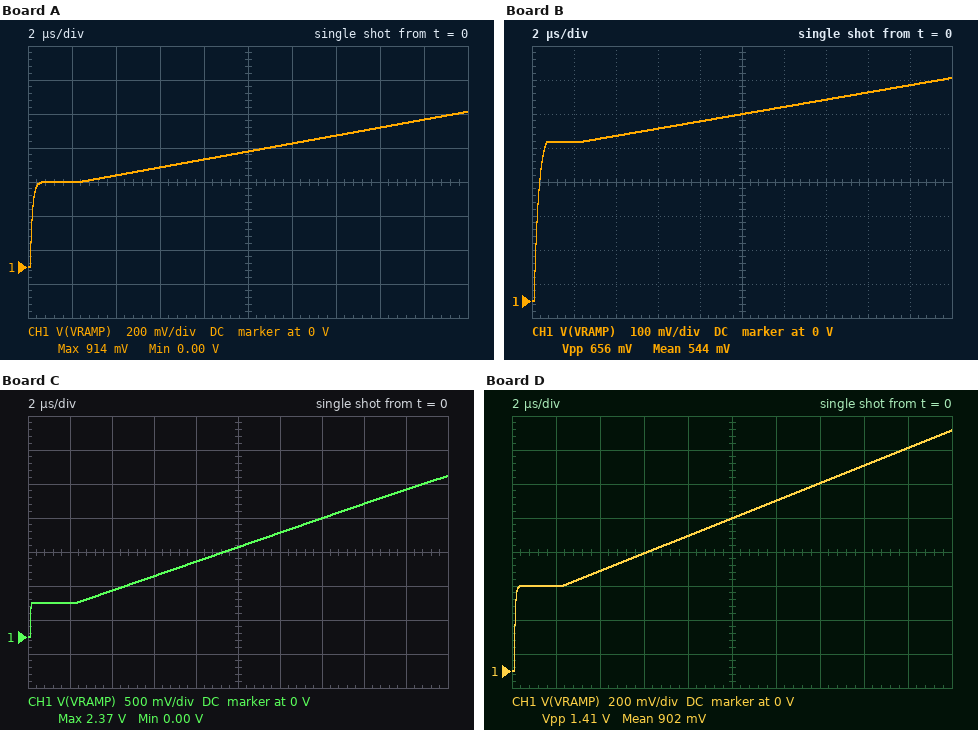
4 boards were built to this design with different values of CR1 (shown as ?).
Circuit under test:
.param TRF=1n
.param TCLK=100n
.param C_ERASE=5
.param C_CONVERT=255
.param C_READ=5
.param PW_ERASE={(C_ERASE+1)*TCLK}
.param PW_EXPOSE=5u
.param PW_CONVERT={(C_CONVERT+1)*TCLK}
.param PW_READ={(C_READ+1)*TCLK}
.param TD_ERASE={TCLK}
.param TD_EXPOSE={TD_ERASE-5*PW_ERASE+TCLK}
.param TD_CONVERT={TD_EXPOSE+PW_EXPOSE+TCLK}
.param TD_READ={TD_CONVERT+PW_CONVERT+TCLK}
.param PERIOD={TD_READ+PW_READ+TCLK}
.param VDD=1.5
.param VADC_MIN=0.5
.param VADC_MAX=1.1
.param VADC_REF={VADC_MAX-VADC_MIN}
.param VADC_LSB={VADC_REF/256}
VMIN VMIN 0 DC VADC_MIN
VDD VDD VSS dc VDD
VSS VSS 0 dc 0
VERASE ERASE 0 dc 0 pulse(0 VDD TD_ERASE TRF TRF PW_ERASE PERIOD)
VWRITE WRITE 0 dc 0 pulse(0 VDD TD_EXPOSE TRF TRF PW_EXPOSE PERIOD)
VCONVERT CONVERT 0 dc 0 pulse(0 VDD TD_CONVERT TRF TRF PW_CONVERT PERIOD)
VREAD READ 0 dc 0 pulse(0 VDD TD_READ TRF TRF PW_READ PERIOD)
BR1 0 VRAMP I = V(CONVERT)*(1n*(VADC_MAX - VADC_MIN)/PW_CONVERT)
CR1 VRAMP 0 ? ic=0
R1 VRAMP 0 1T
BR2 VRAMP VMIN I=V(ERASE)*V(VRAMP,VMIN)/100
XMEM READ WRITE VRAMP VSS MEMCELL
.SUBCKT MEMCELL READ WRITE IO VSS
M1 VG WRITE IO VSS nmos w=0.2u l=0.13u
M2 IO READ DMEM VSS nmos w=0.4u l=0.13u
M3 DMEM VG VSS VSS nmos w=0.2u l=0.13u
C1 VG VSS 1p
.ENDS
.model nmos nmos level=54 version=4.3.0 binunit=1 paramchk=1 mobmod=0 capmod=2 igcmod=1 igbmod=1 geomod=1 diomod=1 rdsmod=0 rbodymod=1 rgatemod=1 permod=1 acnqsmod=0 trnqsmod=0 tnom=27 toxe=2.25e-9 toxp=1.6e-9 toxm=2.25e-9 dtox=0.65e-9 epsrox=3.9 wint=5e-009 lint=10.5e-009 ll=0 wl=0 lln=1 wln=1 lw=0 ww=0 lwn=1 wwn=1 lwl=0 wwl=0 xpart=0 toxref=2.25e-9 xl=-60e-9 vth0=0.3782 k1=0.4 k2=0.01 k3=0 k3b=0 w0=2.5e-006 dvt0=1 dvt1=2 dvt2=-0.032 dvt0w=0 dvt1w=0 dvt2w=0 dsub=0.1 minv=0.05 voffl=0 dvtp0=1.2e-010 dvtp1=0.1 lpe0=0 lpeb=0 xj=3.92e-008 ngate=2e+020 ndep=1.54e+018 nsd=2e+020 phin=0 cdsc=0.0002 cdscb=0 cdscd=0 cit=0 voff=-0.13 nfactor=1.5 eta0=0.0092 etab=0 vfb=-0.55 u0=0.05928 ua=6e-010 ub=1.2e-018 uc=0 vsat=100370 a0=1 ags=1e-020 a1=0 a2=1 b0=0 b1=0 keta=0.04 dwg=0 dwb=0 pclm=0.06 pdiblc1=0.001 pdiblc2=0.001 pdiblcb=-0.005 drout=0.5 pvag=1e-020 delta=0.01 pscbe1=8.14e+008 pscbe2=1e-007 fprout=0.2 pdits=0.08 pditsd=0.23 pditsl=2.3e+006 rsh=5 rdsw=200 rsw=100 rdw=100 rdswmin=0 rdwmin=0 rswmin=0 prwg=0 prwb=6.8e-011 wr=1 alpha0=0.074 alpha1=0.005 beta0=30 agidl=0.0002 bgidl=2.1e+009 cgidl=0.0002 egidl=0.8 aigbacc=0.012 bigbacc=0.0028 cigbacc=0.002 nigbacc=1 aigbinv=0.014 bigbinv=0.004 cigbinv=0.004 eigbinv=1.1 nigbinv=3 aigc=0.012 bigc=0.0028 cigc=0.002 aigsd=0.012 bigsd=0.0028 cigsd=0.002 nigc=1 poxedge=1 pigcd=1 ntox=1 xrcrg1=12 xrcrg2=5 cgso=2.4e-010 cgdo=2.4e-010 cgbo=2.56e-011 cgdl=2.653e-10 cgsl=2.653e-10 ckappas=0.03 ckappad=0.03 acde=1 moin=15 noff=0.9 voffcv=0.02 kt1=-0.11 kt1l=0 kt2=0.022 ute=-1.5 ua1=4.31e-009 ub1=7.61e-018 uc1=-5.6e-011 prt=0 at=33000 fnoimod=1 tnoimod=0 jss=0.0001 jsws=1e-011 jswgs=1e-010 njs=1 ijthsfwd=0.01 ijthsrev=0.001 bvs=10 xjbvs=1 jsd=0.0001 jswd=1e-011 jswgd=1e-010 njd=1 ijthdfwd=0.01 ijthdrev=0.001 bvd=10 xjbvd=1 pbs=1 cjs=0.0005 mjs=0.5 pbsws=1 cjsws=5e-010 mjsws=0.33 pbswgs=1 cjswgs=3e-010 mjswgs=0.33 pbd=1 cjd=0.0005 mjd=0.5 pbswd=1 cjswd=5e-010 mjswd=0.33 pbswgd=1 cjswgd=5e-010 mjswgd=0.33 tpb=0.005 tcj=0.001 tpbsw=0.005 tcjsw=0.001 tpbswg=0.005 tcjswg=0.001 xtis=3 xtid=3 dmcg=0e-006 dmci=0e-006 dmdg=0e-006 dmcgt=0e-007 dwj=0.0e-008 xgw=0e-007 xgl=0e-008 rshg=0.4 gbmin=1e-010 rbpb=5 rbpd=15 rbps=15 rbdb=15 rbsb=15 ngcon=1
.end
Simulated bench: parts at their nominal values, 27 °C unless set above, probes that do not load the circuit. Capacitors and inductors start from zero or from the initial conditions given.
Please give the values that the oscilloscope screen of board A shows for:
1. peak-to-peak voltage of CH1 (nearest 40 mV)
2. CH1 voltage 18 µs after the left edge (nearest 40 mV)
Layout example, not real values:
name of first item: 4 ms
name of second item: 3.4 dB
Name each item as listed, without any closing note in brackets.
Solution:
peak-to-peak voltage of CH1: 920 mV
CH1 voltage 18 µs after the left edge: 880 mV
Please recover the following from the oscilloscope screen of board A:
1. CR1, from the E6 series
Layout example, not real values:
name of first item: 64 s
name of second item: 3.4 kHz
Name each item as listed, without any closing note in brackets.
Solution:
CR1, from the E6 series: 1.5 nF
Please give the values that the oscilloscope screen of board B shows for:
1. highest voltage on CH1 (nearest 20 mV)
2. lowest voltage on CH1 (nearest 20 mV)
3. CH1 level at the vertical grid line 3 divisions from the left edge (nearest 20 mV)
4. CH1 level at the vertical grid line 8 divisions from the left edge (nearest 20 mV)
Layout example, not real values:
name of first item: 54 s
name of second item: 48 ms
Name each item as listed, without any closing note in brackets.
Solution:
highest voltage on CH1: 660 mV
lowest voltage on CH1: 0 V
CH1 level at the vertical grid line 3 divisions from the left edge: 500 mV
CH1 level at the vertical grid line 8 divisions from the left edge: 620 mV
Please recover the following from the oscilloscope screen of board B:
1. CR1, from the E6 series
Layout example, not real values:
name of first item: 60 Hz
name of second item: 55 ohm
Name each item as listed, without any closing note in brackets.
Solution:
CR1, from the E6 series: 3.3 nF
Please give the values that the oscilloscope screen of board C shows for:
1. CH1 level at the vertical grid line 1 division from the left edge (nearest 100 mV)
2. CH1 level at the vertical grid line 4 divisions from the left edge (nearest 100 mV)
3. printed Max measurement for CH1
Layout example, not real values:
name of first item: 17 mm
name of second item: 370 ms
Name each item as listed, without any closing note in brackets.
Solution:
CH1 level at the vertical grid line 1 division from the left edge: 500 mV
CH1 level at the vertical grid line 4 divisions from the left edge: 1.1 V
printed Max measurement for CH1: 2.37 V
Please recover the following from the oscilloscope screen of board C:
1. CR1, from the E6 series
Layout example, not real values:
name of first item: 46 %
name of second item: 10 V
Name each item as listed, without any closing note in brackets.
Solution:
CR1, from the E6 series: 330 pF
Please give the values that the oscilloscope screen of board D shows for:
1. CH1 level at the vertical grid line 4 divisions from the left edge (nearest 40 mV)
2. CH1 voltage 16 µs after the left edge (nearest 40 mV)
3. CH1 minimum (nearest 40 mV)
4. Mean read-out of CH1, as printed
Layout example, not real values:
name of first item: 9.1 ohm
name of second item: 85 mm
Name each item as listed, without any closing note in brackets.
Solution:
CH1 level at the vertical grid line 4 divisions from the left edge: 800 mV
CH1 voltage 16 µs after the left edge: 1.20 V
CH1 minimum: 0 V
Mean read-out of CH1, as printed: 902 mV
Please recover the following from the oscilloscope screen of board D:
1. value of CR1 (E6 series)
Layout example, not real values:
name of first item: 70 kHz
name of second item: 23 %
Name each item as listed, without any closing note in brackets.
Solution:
value of CR1: 680 pF
